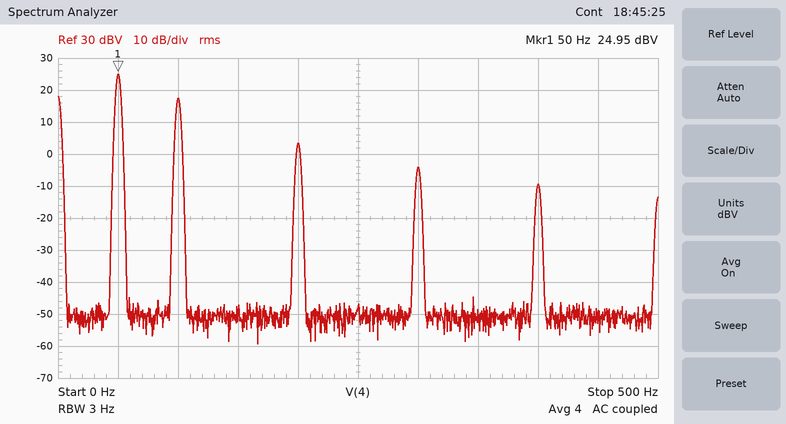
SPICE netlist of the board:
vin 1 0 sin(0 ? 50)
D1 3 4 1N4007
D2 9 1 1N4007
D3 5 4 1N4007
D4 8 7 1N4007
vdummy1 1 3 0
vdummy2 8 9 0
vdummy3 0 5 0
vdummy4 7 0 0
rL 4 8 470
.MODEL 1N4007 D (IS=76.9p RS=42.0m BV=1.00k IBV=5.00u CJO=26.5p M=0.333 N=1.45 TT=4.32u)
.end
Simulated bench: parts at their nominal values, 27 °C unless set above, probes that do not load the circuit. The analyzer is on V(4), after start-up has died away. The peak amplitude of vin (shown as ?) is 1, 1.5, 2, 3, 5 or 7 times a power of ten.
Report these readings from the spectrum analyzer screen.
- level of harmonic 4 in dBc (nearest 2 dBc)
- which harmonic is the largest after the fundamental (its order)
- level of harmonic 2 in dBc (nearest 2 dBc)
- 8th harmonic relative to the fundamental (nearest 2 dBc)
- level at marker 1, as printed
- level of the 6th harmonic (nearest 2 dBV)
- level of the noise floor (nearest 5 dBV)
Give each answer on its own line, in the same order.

-22 dBc
2
-8 dBc
-34 dBc
24.95 dBV
-4 dBV
-50 dBV
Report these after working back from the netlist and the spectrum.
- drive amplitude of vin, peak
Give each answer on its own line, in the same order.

50 V
